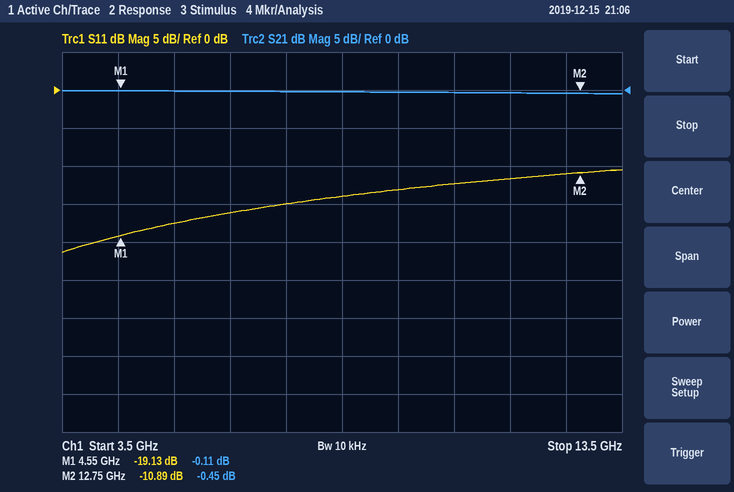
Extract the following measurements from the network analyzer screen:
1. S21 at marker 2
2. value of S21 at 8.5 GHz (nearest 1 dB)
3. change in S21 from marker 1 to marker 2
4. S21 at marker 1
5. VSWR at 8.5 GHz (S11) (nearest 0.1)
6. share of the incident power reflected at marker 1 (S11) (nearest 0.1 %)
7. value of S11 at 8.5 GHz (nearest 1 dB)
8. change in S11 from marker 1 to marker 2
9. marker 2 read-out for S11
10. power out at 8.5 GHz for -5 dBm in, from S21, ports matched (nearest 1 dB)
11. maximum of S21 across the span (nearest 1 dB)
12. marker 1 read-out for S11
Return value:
-0.45 dB
0 dB
-0.34 dB
-0.11 dB
1.5
1.2 %
-14 dB
8.24 dB
-10.89 dB
-5 dBm
0 dB
-19.13 dB
